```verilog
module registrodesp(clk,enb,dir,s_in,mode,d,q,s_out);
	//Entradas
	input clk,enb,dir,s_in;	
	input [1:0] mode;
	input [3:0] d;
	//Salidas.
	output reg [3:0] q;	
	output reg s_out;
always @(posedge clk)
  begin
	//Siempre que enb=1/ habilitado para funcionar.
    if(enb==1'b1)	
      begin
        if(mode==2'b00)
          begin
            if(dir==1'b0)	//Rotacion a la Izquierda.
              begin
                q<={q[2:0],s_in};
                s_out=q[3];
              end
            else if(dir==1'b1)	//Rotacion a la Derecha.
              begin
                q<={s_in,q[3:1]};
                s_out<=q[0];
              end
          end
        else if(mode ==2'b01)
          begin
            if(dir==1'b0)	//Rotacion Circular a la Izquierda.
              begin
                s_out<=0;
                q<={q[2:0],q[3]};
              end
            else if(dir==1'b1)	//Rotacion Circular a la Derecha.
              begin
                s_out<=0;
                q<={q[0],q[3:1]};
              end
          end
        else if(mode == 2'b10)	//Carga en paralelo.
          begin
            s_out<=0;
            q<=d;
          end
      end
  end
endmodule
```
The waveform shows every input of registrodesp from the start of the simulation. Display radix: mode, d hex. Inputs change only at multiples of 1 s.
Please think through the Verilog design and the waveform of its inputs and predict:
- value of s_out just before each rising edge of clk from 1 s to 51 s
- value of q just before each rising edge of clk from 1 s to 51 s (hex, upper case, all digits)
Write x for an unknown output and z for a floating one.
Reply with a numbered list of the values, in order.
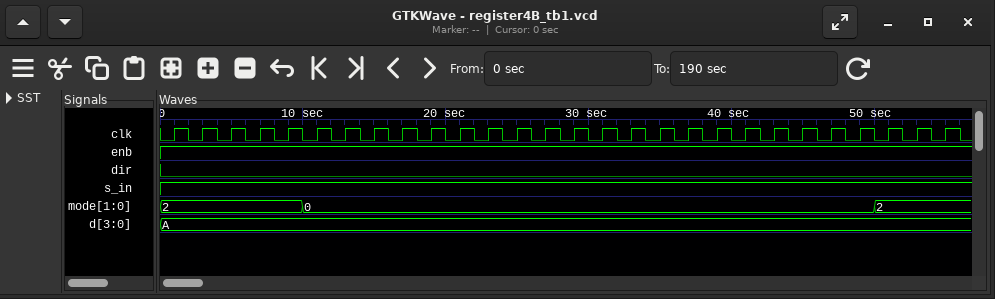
1. x 0 0 0 0 0 1 0 1 0 1 1 1 1 1 1 1 1 1 1 1 1 1 1 1 1
2. x, A, A, A, A, A, 5, B, 7, F, F, F, F, F, F, F, F, F, F, F, F, F, F, F, F, F
